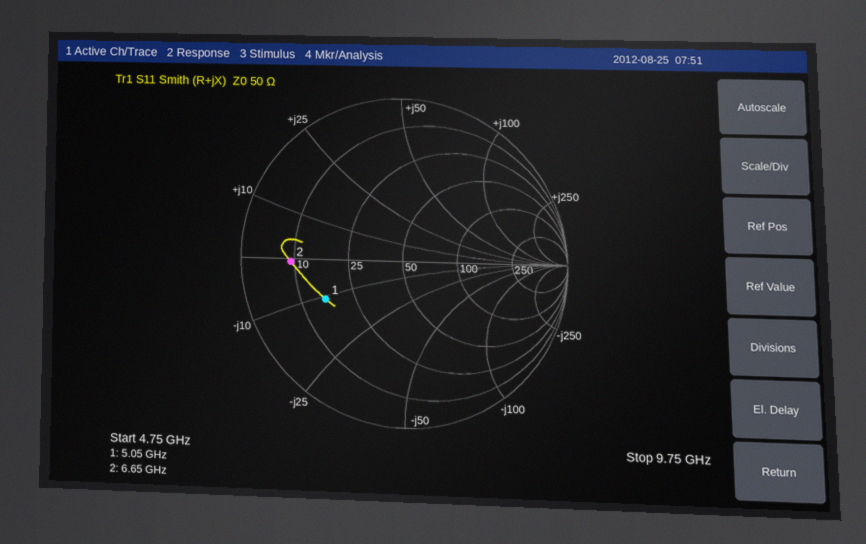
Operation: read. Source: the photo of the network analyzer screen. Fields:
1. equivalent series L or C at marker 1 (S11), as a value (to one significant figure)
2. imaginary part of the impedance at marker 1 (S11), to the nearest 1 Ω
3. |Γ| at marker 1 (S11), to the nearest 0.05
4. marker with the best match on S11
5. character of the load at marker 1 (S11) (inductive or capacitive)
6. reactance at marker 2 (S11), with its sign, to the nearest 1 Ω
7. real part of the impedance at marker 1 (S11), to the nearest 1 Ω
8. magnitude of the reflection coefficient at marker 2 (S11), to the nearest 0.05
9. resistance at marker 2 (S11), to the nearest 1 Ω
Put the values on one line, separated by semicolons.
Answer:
3 pF; -11 Ω; 0.55; marker 1; capacitive; -1 Ω; 16 Ω; 0.70; 9 Ω
